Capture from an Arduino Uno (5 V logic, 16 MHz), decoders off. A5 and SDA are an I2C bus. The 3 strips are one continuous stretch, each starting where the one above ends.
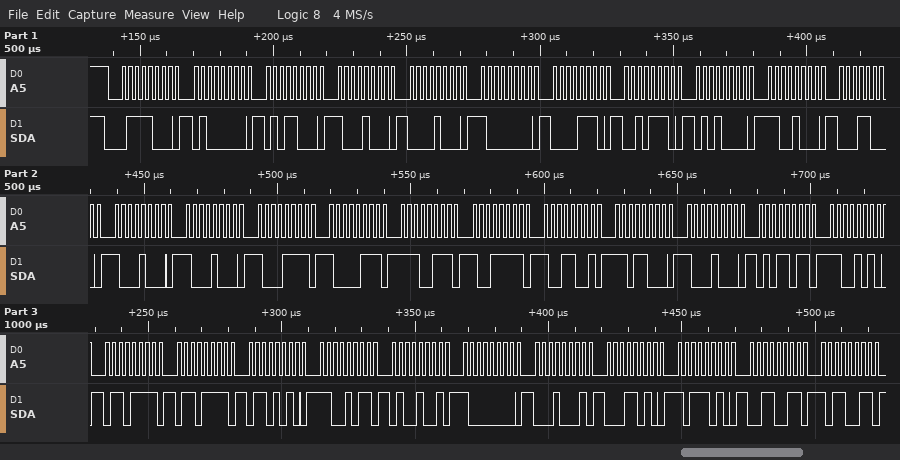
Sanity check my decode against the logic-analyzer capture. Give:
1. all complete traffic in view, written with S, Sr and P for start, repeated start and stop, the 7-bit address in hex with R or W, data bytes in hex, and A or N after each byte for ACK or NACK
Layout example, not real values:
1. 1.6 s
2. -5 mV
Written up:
1. S 3CW A 40 A 58 A 88 A 08 A 80 A 0E A 2E A 50 A C8 A 18 A 88 A 88 A 8F A 87 A E7 A 9F A 99 A D8 A 88 A 5B A CA A 6F A 6F A 6A A CB A 49 A 80 A 11 A 1A A BA A 33 A B3 A
